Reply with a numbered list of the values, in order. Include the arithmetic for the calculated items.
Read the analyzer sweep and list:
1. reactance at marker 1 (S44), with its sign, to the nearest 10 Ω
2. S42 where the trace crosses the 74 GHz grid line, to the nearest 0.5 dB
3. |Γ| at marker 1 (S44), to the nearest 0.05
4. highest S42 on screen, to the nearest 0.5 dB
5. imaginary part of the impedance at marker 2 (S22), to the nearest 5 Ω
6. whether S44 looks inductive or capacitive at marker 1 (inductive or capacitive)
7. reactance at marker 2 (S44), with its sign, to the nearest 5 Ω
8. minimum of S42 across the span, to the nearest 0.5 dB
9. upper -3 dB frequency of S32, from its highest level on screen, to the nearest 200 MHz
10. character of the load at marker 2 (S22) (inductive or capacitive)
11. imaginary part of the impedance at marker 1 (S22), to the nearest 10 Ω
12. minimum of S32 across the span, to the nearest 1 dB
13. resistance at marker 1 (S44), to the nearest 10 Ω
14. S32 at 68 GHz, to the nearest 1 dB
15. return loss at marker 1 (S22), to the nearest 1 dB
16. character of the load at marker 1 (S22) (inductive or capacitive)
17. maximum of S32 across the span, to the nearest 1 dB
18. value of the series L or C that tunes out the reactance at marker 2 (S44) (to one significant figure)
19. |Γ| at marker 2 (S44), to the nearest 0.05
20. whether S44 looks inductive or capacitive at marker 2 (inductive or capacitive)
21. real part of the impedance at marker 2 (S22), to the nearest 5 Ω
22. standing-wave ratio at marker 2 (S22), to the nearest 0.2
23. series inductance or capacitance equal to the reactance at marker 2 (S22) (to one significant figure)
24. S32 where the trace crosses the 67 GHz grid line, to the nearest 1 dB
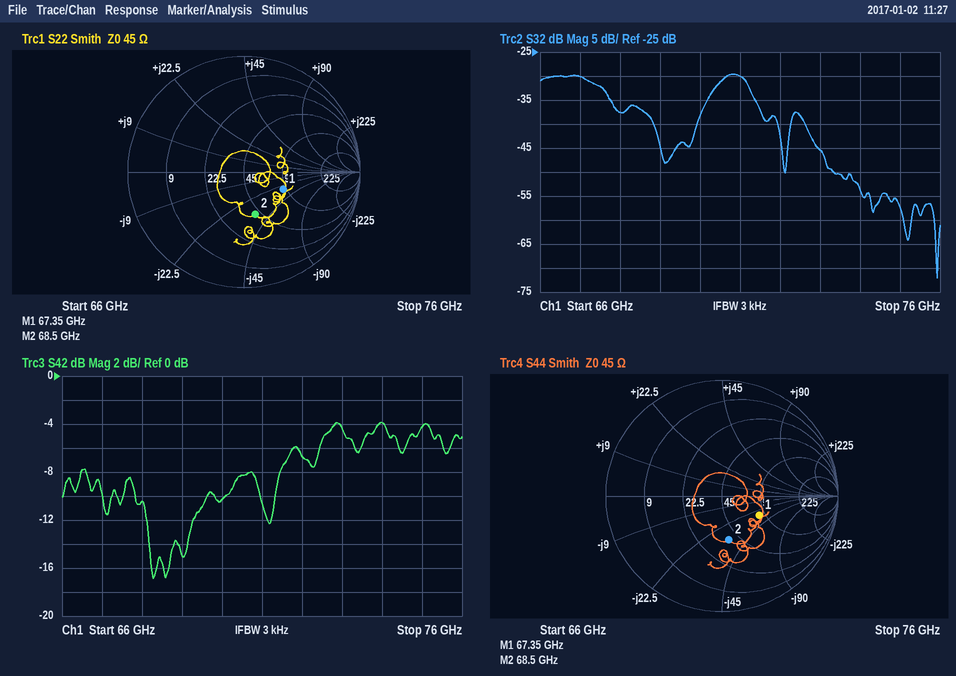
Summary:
1. -30 Ω
2. -4.0 dB
3. 0.35
4. -4.0 dB
5. -35 Ω
6. capacitive
7. -35 Ω
8. -17.0 dB
9. 71.2 GHz
10. capacitive
11. -30 Ω
12. -72 dB
13. 80 Ω
14. -38 dB
15. 9 dB
16. capacitive
17. -30 dB
18. L = 35 Ω/(2π × 68.5 GHz) ≈ 81.3 pH, so 80 pH to one significant figure
19. 0.40
20. capacitive
21. 40 Ω
22. 2.2
23. C = 1/(2π × 68.5 GHz × 35 Ω) ≈ 66.4 fF, so 70 fF to one significant figure
24. -30 dB
